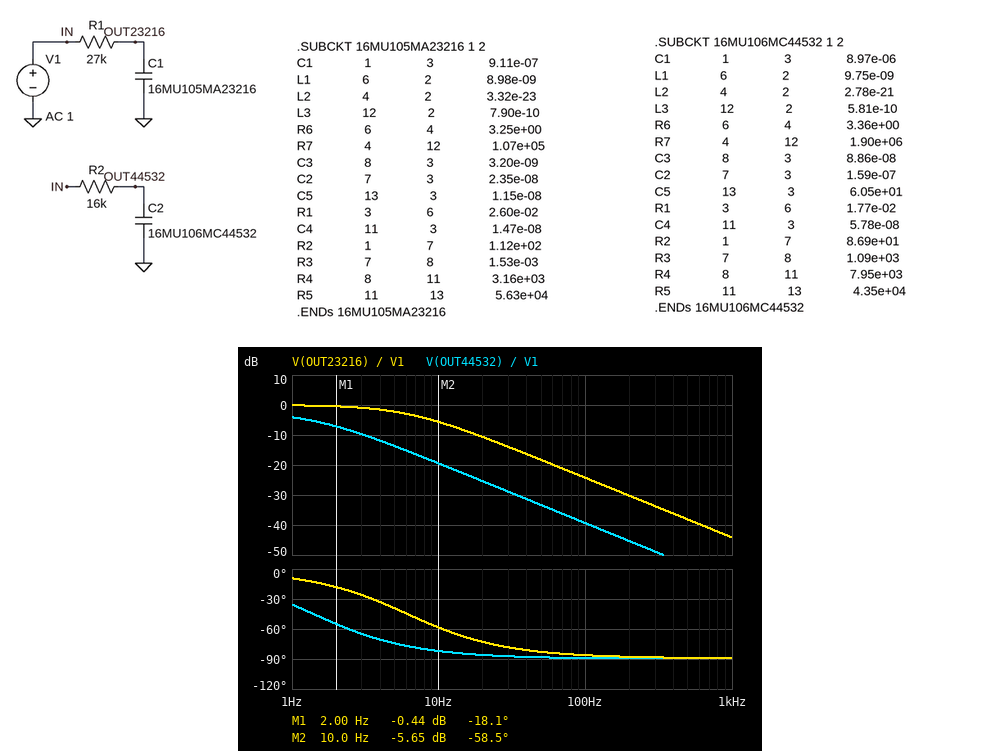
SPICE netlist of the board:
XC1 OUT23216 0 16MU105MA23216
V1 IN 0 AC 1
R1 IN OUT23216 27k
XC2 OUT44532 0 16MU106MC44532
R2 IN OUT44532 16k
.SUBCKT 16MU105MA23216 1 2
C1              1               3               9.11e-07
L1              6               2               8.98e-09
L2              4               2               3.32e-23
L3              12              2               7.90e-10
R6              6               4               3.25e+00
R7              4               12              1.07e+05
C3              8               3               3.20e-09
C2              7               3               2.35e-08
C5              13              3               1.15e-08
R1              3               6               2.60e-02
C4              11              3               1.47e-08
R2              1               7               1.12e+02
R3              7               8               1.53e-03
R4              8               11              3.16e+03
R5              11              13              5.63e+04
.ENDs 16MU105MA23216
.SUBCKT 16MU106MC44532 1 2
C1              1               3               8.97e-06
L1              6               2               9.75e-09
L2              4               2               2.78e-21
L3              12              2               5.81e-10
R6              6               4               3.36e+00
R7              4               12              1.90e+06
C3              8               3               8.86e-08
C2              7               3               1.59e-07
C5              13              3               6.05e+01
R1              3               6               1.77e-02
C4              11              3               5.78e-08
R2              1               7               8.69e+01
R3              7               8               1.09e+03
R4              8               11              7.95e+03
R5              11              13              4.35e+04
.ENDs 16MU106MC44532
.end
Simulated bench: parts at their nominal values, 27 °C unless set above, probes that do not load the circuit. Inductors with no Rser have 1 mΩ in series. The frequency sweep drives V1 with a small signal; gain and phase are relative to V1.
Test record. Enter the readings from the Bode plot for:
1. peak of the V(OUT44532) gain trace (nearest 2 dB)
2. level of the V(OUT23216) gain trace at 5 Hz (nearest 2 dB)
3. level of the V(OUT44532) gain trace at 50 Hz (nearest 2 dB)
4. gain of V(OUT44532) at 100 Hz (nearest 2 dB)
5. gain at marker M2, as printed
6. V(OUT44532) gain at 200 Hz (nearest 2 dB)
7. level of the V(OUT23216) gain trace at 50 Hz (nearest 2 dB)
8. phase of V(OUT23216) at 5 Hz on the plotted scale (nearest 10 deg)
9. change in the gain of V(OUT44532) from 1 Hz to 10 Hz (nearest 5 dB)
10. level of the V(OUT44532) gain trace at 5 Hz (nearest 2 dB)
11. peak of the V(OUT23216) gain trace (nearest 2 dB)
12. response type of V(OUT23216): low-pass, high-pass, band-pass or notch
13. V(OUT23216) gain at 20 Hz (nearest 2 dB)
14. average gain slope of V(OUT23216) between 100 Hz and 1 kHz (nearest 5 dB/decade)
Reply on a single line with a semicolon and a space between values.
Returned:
-4 dB; -2 dB; -34 dB; -40 dB; -5.65 dB; -46 dB; -18 dB; -40 deg; -15 dB; -14 dB; 0 dB; low-pass; -10 dB; -20 dB/decade
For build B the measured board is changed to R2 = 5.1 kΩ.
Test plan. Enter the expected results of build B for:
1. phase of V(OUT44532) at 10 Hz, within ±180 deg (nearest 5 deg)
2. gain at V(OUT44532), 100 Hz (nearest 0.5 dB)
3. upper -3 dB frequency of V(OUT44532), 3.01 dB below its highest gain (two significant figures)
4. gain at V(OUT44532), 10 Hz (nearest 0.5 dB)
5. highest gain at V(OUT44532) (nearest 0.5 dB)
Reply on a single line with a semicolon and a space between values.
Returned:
-70 deg; -29.5 dB; 3.7 Hz; -10.0 dB; -1.0 dB
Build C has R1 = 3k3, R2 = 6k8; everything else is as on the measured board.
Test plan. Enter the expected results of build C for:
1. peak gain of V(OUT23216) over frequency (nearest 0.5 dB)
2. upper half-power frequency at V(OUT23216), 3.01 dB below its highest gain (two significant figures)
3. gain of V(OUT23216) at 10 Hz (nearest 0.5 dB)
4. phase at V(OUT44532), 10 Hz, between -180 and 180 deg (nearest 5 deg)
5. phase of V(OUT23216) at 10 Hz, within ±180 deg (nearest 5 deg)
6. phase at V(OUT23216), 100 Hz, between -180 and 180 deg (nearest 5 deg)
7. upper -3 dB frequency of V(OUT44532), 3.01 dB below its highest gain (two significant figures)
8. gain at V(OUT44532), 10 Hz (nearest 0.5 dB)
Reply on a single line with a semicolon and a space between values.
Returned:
0 dB; 50 Hz; 0 dB; -75 deg; -10 deg; -65 deg; 2.9 Hz; -12.5 dB
